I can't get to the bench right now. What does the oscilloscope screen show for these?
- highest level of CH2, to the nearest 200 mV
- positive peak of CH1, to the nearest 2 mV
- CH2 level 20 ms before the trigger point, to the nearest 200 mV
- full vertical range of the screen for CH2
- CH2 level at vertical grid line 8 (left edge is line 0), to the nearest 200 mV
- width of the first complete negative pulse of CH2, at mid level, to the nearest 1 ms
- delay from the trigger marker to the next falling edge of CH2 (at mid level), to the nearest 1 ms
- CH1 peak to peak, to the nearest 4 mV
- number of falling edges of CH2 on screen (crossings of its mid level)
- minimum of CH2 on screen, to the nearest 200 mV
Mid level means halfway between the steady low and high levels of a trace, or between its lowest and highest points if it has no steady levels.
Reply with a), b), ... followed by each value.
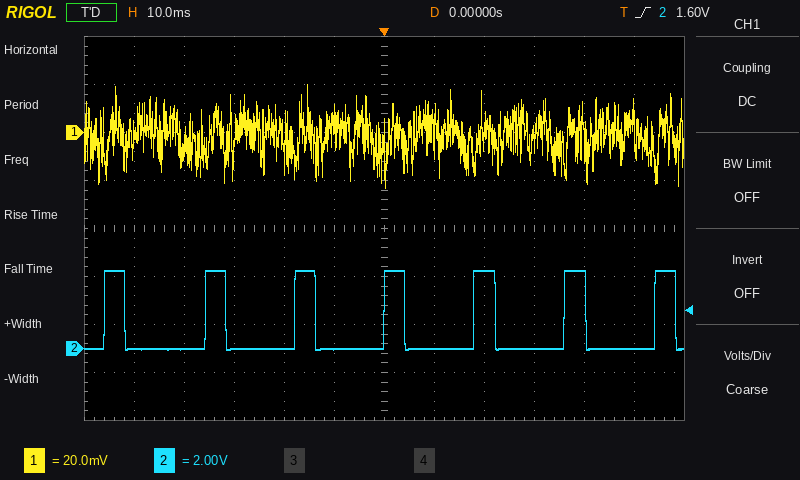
a) 3.2 V
b) 20 mV
c) 0.0 V
d) 16 V
e) 3.2 V
f) 16 ms
g) 4 ms
h) 44 mV
i) 7
j) 0.0 V
